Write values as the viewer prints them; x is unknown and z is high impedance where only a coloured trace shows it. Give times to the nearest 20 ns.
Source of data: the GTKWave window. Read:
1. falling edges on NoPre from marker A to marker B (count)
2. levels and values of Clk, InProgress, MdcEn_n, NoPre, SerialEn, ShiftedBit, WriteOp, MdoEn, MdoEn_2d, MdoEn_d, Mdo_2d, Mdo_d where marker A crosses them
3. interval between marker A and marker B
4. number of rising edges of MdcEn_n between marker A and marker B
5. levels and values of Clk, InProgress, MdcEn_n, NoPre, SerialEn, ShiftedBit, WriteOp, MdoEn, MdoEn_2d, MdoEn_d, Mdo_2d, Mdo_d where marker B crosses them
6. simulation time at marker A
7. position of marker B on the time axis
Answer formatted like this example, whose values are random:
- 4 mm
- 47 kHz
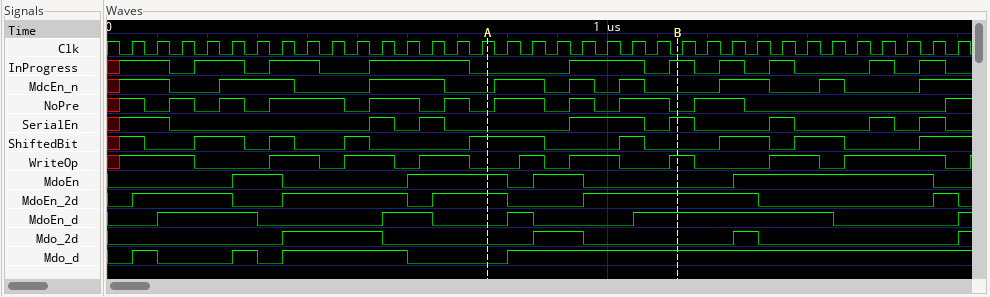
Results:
- 3
- Clk=1, InProgress=0, MdcEn_n=0, NoPre=0, SerialEn=0, ShiftedBit=1, WriteOp=0, MdoEn=1, MdoEn_2d=1, MdoEn_d=0, Mdo_2d=0, Mdo_d=0
- 380 ns
- 3
- Clk=0, InProgress=1, MdcEn_n=0, NoPre=0, SerialEn=1, ShiftedBit=0, WriteOp=1, MdoEn=0, MdoEn_2d=1, MdoEn_d=1, Mdo_2d=0, Mdo_d=1
- 760 ns
- 1140 ns
